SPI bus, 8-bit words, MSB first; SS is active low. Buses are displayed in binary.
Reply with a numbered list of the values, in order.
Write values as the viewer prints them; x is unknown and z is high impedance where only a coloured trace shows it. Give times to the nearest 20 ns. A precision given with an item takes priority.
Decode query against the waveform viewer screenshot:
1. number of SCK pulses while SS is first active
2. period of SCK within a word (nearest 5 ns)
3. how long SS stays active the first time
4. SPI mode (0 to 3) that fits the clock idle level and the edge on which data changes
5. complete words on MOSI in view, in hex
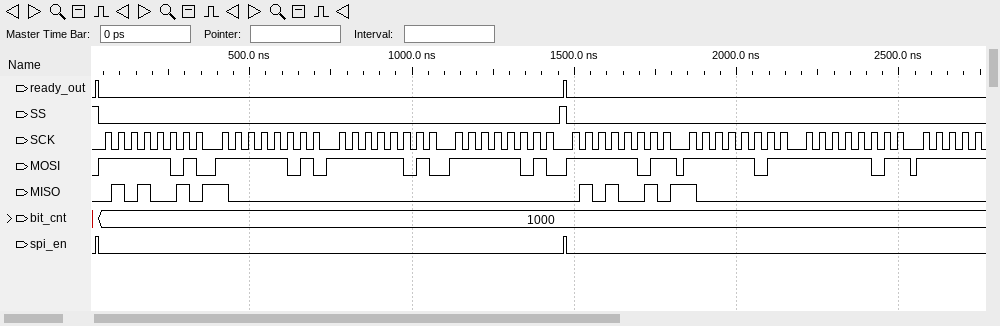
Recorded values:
1. 32
2. 40 ns
3. 1420 ns
4. 1
5. FA, FA, FA, FA, FB, FB, FB
